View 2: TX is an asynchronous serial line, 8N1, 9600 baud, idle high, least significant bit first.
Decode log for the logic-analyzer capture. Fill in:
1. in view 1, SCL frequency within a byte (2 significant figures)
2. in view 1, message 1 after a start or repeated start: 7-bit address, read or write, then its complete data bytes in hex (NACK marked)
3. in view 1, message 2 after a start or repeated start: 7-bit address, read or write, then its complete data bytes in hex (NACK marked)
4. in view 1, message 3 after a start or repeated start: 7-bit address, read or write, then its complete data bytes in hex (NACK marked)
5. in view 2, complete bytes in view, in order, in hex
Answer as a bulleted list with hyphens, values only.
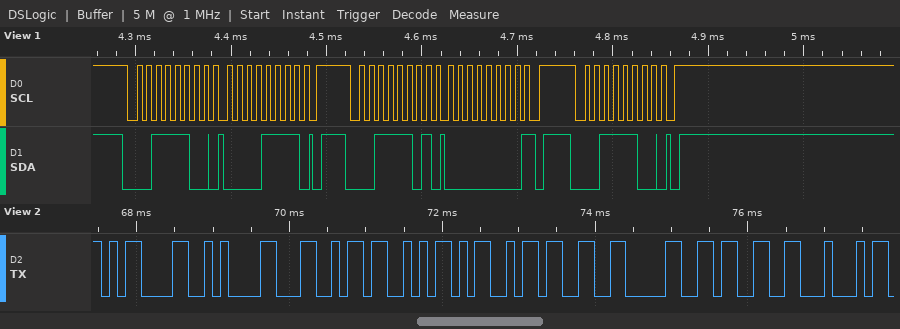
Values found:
- 100 kHz
- 0x1E write: 0F
- 0x1E read: 00 NACK
- 0x1E write
- 0D 0A 4C 53 4D 33 30 33 44
